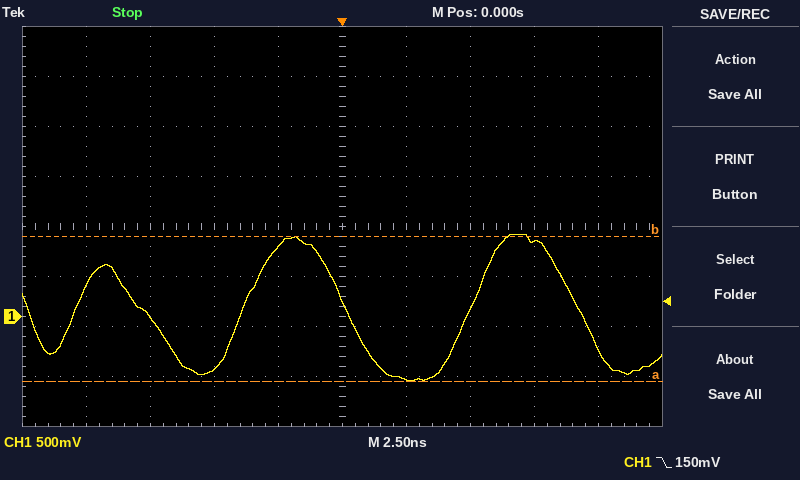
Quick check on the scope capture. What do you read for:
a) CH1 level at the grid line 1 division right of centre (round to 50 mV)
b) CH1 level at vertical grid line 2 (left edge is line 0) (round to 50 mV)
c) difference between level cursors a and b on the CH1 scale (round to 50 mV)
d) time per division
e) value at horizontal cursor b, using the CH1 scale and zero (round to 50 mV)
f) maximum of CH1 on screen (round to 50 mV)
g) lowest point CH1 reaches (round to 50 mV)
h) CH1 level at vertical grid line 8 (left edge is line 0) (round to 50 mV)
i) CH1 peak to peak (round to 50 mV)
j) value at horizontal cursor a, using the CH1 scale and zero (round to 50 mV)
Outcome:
-650 mV
0 mV
1.45 V
2.5 ns
800 mV
800 mV
-650 mV
750 mV
1.45 V
-650 mV
